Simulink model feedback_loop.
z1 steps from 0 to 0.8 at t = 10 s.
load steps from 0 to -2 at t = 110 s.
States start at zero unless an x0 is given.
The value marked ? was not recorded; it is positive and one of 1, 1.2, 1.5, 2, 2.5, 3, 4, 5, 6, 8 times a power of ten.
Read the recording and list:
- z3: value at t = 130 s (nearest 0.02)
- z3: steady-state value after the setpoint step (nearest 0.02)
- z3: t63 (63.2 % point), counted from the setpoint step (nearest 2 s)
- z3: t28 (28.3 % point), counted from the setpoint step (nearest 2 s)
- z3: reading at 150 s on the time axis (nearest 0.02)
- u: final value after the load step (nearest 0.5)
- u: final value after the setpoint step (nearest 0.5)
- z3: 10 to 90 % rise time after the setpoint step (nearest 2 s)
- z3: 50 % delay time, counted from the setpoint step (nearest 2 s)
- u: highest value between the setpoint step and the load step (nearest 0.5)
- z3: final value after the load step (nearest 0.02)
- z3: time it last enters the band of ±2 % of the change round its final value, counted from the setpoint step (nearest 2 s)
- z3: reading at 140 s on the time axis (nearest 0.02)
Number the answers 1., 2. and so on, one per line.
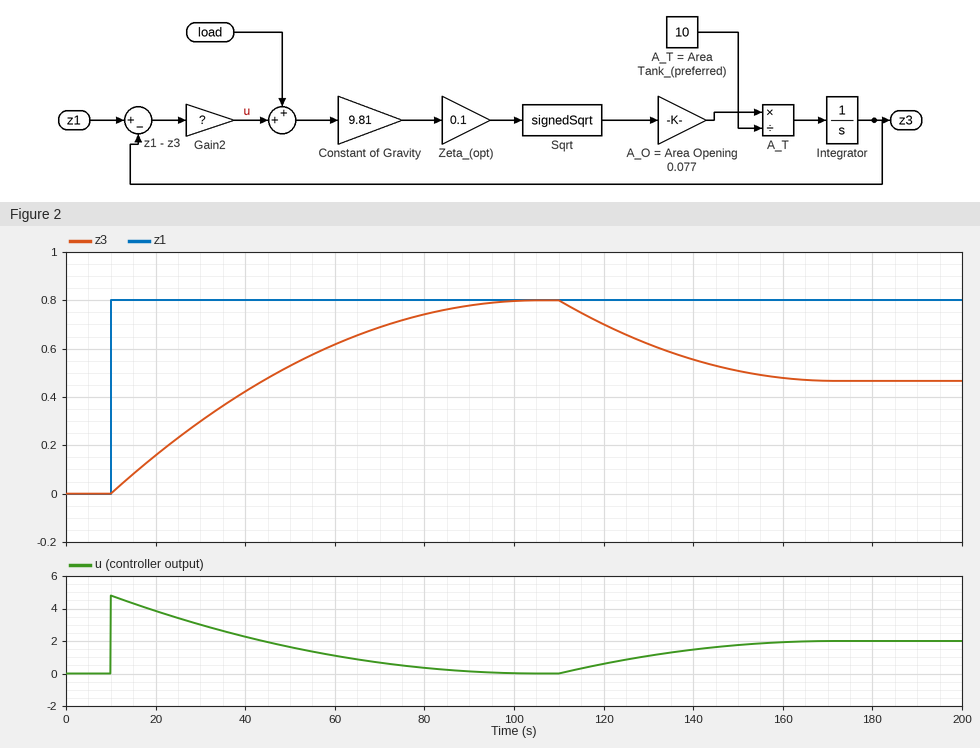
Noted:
1. 0.62
2. 0.80
3. 38 s
4. 14 s
5. 0.50
6. 2.0
7. 0.0
8. 60 s
9. 28 s
10. 5.0
11. 0.46
12. 82 s
13. 0.56
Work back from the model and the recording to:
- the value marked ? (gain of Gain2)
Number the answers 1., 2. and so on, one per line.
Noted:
1. 6
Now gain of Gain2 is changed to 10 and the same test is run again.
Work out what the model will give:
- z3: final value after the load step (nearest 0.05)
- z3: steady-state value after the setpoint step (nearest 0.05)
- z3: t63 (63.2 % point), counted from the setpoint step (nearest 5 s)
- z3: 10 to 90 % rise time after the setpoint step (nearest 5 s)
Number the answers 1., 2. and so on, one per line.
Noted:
1. 0.60
2. 0.80
3. 30 s
4. 45 s
